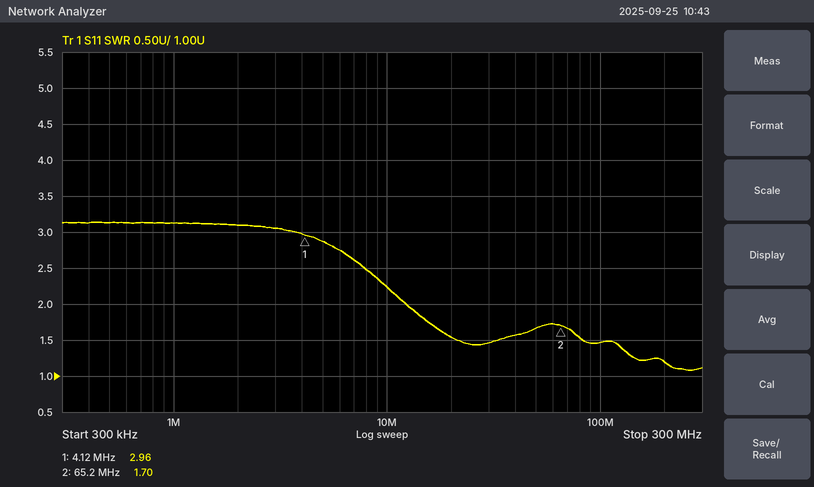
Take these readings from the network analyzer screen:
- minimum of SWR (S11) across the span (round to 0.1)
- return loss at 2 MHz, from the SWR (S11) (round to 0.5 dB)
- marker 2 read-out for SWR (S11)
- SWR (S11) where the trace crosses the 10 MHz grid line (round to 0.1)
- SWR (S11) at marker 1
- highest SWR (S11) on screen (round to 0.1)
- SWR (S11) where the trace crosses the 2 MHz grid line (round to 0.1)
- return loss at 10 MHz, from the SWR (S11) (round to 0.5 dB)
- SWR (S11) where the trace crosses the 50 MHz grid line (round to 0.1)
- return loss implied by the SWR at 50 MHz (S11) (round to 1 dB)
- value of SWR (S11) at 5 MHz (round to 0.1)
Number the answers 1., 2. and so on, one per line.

1. 1.1
2. 6.0 dB
3. 1.70
4. 2.2
5. 2.96
6. 3.1
7. 3.1
8. 8.5 dB
9. 1.7
10. 12 dB
11. 2.9
